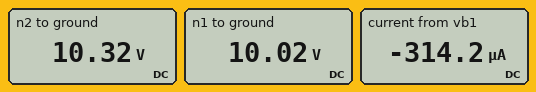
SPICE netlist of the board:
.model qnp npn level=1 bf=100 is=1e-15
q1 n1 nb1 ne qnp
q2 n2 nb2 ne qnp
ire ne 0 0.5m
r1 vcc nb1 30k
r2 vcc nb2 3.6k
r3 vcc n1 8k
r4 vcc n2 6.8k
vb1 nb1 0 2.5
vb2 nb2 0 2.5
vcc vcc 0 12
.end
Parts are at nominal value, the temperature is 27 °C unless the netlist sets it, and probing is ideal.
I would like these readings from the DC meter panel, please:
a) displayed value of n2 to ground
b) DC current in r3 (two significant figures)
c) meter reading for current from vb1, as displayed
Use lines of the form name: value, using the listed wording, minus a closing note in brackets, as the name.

displayed value of n2 to ground: 10.32 V
DC current in r3: 250 µA
meter reading for current from vb1, as displayed: -314.2 µA
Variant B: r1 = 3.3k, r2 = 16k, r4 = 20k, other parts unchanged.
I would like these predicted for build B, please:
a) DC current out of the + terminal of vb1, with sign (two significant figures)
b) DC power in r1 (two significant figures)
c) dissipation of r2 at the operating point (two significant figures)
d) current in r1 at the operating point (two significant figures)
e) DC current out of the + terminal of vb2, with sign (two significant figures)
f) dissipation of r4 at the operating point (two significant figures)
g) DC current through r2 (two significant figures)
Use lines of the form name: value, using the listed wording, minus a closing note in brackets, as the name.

DC current out of the + terminal of vb1, with sign: -2.9 mA
DC power in r1: 27 mW
dissipation of r2 at the operating point: 5.6 mW
current in r1 at the operating point: 2.9 mA
DC current out of the + terminal of vb2, with sign: -590 µA
dissipation of r4 at the operating point: 1.2 mW
DC current through r2: 590 µA
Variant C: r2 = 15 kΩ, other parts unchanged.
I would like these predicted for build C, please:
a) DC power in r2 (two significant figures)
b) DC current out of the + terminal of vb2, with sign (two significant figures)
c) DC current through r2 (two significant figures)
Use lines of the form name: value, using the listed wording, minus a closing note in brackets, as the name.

DC power in r2: 6.0 mW
DC current out of the + terminal of vb2, with sign: -630 µA
DC current through r2: 630 µA
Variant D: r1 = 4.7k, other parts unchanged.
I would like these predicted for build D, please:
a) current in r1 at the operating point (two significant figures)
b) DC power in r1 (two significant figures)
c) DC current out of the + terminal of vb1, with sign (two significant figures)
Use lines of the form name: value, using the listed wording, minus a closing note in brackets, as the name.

current in r1 at the operating point: 2.0 mA
DC power in r1: 19 mW
DC current out of the + terminal of vb1, with sign: -2.0 mA
